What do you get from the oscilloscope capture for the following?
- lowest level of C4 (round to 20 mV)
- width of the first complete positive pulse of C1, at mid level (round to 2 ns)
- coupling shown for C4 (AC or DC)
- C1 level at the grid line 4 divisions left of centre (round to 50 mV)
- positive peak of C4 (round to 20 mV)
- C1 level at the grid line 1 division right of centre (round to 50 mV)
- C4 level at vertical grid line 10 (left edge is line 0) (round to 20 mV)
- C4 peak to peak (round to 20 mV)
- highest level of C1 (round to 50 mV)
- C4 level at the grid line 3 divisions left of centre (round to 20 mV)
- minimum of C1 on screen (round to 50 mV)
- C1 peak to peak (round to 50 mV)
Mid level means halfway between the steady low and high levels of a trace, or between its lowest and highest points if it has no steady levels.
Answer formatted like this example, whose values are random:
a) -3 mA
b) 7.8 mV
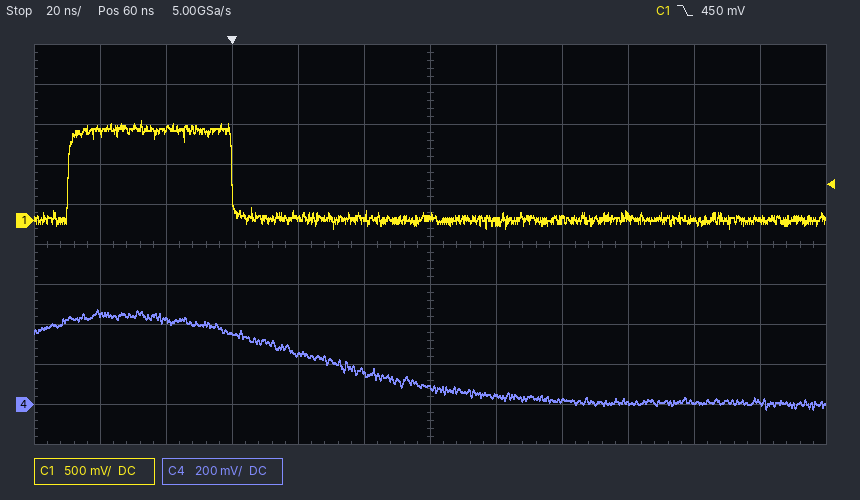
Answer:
a) -20 mV
b) 50 ns
c) DC
d) 1.15 V
e) 480 mV
f) 0 mV
g) 20 mV
h) 500 mV
i) 1.25 V
j) 360 mV
k) -100 mV
l) 1.35 V
